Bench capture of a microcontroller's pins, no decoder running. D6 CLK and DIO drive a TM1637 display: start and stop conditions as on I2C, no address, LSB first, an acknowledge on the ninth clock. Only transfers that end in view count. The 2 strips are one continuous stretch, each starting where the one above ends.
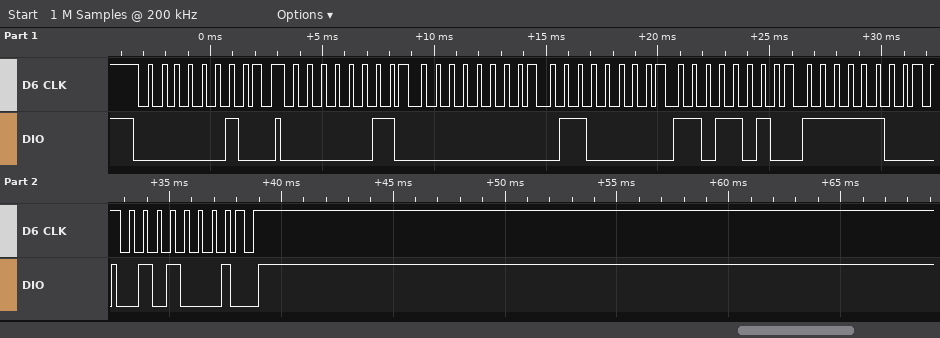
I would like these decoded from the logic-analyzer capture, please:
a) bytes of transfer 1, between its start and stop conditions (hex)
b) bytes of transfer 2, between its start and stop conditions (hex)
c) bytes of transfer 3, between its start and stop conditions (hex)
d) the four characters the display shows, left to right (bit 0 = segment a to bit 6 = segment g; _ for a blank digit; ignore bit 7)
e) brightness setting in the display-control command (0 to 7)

40
C0 00 06 5B 3F
8A
_120
2
